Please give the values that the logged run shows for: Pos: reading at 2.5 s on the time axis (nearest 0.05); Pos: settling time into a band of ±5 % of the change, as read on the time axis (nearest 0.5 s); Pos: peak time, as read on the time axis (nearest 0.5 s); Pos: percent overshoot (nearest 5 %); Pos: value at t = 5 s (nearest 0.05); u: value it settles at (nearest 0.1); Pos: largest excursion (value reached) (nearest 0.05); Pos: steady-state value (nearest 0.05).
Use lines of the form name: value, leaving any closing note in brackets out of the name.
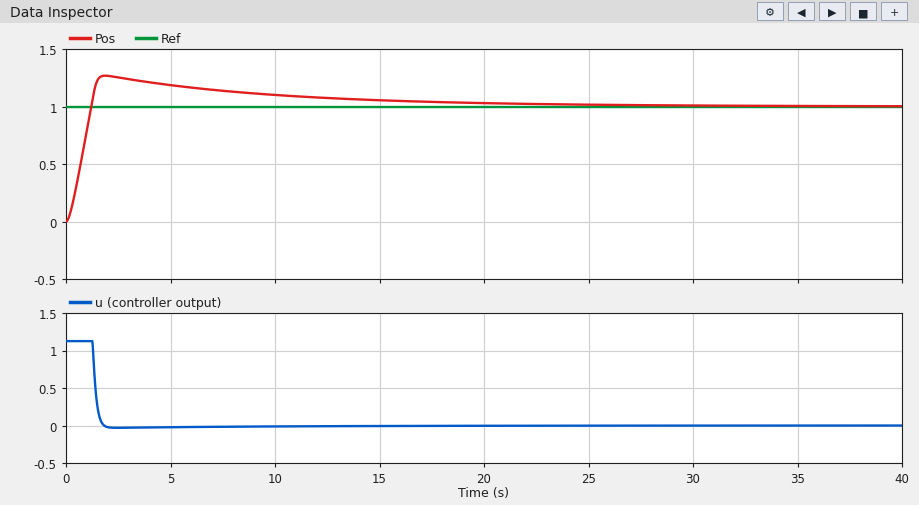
Pos: reading at 2.5 s on the time axis: 1.25
Pos: settling time into a band of ±5 % of the change, as read on the time axis: 15.5 s
Pos: peak time, as read on the time axis: 2.0 s
Pos: percent overshoot: 25 %
Pos: value at t = 5 s: 1.20
u: value it settles at: 0.0
Pos: largest excursion (value reached): 1.25
Pos: steady-state value: 1.00
